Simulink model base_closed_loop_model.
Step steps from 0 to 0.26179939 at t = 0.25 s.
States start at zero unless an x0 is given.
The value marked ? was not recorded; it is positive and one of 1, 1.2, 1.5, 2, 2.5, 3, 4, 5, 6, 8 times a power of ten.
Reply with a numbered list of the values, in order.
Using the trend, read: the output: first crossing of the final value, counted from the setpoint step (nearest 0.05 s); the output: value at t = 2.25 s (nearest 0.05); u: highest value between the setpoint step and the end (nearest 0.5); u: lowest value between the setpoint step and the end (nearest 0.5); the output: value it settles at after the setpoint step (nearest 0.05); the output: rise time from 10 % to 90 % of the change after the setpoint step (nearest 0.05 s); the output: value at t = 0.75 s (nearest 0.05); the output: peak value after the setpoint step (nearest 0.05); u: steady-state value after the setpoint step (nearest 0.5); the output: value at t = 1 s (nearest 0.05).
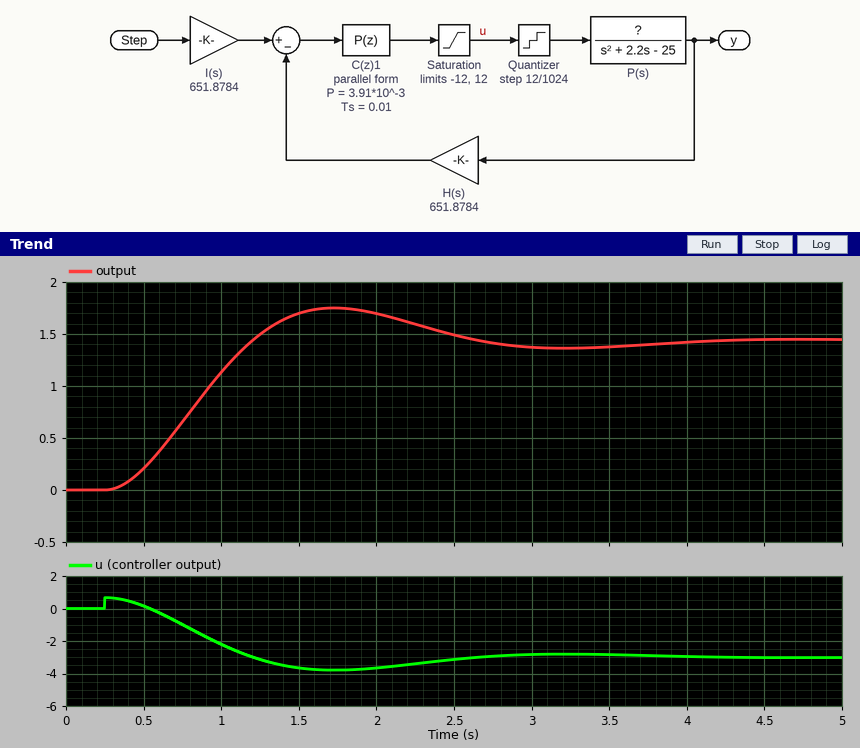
1. 0.95 s
2. 1.60
3. 0.5
4. -4.0
5. 1.45
6. 0.65 s
7. 0.65
8. 1.75
9. -3.0
10. 1.15
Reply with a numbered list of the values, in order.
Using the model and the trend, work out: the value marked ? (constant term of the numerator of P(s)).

1. 12
